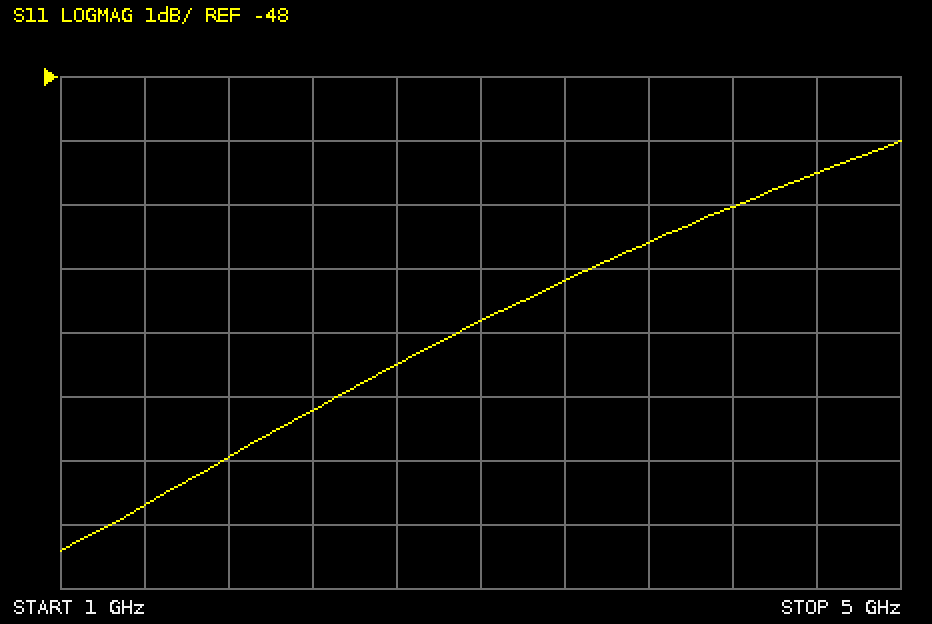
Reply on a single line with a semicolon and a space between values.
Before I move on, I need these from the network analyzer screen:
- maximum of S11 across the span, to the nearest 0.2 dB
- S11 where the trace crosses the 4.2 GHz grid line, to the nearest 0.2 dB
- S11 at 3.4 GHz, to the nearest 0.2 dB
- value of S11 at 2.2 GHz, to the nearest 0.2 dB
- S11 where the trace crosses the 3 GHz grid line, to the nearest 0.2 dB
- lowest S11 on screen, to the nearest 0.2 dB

-49.0 dB; -50.0 dB; -51.2 dB; -53.2 dB; -51.8 dB; -55.4 dB
